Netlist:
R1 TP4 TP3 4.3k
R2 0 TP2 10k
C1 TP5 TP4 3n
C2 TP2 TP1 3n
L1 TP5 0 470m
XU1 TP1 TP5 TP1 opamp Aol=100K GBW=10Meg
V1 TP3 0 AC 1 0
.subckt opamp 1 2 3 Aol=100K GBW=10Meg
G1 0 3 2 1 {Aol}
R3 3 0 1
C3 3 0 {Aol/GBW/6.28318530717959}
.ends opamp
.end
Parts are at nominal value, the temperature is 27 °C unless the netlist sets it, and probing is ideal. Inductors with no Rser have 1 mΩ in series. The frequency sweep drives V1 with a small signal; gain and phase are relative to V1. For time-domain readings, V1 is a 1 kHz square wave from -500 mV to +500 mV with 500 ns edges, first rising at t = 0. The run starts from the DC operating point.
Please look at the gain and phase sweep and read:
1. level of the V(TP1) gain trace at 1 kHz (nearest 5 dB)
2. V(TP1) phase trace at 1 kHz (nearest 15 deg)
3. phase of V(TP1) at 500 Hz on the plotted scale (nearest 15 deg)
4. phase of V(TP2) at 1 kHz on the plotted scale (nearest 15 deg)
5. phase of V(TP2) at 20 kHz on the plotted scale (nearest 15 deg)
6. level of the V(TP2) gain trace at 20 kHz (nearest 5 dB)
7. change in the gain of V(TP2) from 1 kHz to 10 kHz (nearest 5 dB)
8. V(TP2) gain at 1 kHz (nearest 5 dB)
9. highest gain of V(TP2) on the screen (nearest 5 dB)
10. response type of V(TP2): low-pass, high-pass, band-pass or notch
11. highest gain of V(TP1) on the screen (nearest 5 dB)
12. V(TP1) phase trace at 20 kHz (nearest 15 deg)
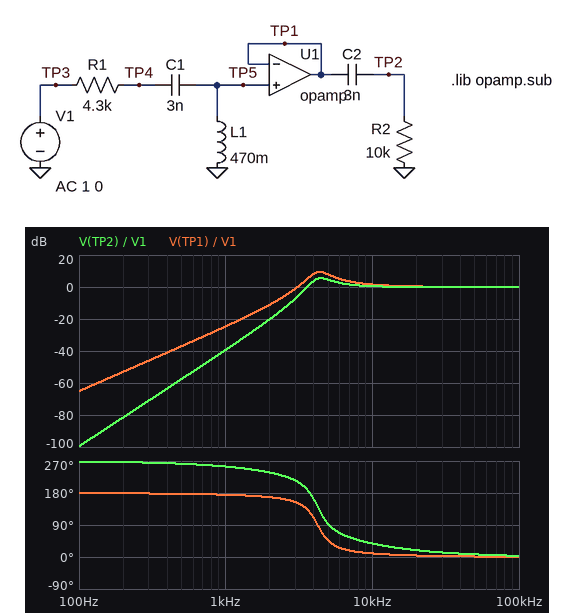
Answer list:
-25 dB
180 deg
180 deg
255 deg
15 deg
0 dB
40 dB
-40 dB
5 dB
high-pass
10 dB
0 deg
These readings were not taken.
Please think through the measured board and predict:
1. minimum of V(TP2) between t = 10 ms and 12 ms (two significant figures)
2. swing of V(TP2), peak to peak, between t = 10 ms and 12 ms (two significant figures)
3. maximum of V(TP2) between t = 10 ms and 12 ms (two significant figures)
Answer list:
-1.0 V
2.0 V
1.0 V
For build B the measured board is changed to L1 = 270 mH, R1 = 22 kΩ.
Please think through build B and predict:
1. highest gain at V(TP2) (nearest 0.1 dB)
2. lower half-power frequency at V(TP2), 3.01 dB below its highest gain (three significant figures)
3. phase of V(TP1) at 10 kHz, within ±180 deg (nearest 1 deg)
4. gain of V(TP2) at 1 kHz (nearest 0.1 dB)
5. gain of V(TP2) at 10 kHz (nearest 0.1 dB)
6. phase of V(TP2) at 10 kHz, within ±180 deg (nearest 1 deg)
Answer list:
0 dB
12.6 kHz
62 deg
-45.0 dB
-4.4 dB
90 deg
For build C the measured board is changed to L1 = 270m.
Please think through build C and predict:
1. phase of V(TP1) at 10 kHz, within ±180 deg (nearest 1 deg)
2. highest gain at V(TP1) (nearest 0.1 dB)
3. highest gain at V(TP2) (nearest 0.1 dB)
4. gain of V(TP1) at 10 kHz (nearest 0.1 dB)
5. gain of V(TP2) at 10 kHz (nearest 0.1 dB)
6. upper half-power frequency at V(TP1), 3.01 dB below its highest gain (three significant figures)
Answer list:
20 deg
7.1 dB
4.6 dB
2.7 dB
1.6 dB
8.28 kHz
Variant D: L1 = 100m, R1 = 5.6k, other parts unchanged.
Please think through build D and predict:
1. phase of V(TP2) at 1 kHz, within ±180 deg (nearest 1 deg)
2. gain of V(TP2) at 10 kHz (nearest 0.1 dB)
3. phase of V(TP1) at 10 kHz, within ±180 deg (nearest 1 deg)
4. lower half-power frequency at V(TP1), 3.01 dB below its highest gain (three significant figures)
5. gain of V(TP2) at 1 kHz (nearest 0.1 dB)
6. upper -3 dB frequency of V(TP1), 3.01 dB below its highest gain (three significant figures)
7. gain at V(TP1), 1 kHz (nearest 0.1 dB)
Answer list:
-107 deg
-0.2 dB
80 deg
7.83 kHz
-53.1 dB
6.63 MHz
-38.5 dB
